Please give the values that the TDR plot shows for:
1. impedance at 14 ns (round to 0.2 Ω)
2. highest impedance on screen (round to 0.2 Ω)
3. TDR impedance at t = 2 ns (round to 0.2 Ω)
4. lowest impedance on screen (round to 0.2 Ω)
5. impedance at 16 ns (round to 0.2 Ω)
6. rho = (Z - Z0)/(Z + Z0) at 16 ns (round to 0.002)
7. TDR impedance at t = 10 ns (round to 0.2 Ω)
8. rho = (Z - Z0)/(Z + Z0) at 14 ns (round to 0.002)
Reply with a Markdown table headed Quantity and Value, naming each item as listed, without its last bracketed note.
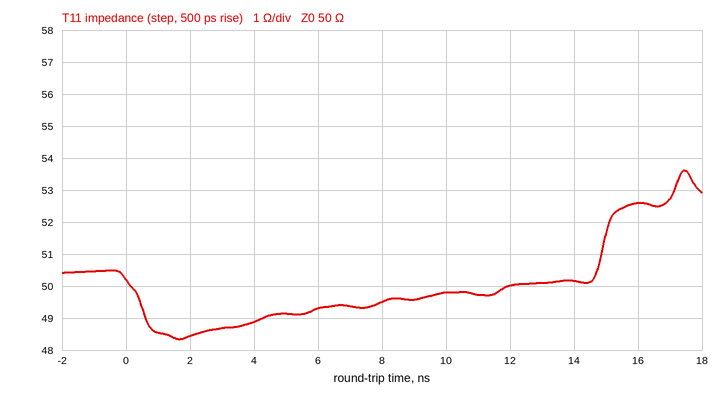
| Quantity | Value |
|---|---|
| impedance at 14 ns | 50.2 Ω |
| highest impedance on screen | 53.6 Ω |
| TDR impedance at t = 2 ns | 48.4 Ω |
| lowest impedance on screen | 48.4 Ω |
| impedance at 16 ns | 52.6 Ω |
| rho = (Z - Z0)/(Z + Z0) at 16 ns | +0.026 |
| TDR impedance at t = 10 ns | 49.8 Ω |
| rho = (Z - Z0)/(Z + Z0) at 14 ns | +0.002 |
